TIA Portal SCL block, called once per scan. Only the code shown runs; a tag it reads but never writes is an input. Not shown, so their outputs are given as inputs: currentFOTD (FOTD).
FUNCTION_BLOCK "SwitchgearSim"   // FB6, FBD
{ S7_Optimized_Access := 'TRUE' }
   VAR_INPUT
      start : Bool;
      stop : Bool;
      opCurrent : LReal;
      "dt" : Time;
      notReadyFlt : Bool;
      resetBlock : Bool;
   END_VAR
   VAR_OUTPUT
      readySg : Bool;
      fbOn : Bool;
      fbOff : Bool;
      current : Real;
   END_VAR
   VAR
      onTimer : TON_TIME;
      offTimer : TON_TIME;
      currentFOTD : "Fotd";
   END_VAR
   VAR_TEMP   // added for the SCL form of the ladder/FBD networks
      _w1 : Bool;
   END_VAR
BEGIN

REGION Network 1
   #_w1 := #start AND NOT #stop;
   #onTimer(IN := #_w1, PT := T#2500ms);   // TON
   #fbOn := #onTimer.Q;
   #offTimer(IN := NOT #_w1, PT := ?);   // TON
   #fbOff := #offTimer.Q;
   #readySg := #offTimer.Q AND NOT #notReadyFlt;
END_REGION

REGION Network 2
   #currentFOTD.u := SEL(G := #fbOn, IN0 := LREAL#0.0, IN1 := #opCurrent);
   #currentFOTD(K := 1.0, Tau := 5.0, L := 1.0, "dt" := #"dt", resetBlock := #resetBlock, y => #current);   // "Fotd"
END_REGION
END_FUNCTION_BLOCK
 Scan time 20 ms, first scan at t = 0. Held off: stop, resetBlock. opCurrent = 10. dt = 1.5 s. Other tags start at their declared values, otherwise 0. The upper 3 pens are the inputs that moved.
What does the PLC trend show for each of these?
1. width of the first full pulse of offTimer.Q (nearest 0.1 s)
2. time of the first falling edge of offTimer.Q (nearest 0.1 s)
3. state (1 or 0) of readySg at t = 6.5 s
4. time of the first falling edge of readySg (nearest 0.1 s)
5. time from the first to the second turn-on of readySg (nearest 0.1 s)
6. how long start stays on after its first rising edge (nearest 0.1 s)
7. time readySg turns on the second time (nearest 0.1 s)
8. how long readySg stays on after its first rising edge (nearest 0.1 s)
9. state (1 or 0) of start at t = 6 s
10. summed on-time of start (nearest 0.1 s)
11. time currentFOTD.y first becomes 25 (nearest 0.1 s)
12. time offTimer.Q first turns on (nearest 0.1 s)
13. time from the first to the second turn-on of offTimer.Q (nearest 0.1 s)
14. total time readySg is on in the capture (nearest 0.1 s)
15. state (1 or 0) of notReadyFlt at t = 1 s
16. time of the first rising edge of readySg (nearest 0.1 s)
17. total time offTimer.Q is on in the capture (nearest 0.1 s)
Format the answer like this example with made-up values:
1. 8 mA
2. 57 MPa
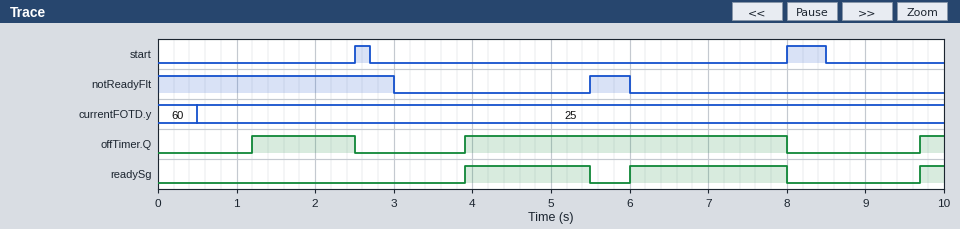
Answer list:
1. 1.3 s
2. 2.5 s
3. 1
4. 5.5 s
5. 2.1 s
6. 0.2 s
7. 6.0 s
8. 1.6 s
9. 0
10. 0.7 s
11. 0.5 s
12. 1.2 s
13. 2.7 s
14. 3.9 s
15. 1
16. 3.9 s
17. 5.7 s
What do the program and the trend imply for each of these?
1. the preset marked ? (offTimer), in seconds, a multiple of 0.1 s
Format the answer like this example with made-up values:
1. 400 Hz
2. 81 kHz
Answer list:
1. 1.2 s
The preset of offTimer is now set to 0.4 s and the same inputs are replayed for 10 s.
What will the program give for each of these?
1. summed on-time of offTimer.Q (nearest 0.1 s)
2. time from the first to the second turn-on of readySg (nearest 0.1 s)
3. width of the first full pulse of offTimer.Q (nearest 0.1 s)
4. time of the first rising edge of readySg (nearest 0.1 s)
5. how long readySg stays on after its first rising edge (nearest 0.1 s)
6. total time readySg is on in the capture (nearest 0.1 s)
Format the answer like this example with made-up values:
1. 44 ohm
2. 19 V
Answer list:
1. 8.1 s
2. 2.9 s
3. 2.1 s
4. 3.1 s
5. 2.4 s
6. 5.5 s
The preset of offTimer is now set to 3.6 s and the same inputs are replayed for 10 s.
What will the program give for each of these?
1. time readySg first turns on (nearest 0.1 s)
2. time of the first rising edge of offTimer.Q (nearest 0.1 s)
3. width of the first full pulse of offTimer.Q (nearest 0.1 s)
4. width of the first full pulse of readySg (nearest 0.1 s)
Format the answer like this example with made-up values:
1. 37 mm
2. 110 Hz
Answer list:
1. 6.3 s
2. 6.3 s
3. 1.7 s
4. 1.7 s
